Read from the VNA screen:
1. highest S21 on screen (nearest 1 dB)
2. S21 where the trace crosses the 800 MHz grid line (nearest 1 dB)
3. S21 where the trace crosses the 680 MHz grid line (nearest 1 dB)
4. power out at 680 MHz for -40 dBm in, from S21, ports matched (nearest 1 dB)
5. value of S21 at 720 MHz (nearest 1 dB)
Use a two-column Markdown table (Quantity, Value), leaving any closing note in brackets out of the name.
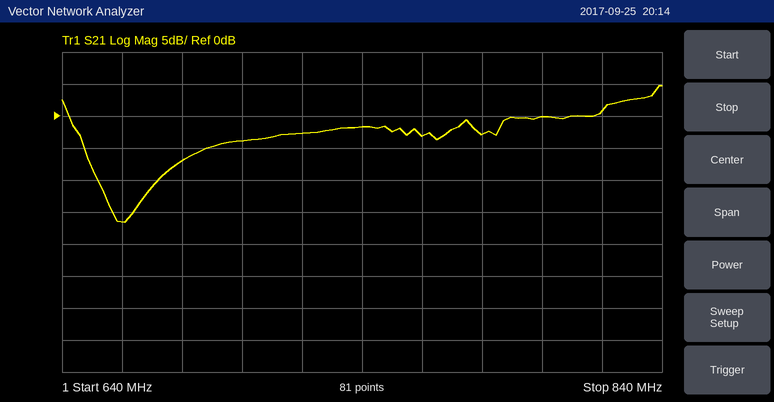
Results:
| Quantity | Value |
|---|---|
| highest S21 on screen | 5 dB |
| S21 where the trace crosses the 800 MHz grid line | 0 dB |
| S21 where the trace crosses the 680 MHz grid line | -7 dB |
| power out at 680 MHz for -40 dBm in, from S21, ports matched | -47 dBm |
| value of S21 at 720 MHz | -3 dB |
